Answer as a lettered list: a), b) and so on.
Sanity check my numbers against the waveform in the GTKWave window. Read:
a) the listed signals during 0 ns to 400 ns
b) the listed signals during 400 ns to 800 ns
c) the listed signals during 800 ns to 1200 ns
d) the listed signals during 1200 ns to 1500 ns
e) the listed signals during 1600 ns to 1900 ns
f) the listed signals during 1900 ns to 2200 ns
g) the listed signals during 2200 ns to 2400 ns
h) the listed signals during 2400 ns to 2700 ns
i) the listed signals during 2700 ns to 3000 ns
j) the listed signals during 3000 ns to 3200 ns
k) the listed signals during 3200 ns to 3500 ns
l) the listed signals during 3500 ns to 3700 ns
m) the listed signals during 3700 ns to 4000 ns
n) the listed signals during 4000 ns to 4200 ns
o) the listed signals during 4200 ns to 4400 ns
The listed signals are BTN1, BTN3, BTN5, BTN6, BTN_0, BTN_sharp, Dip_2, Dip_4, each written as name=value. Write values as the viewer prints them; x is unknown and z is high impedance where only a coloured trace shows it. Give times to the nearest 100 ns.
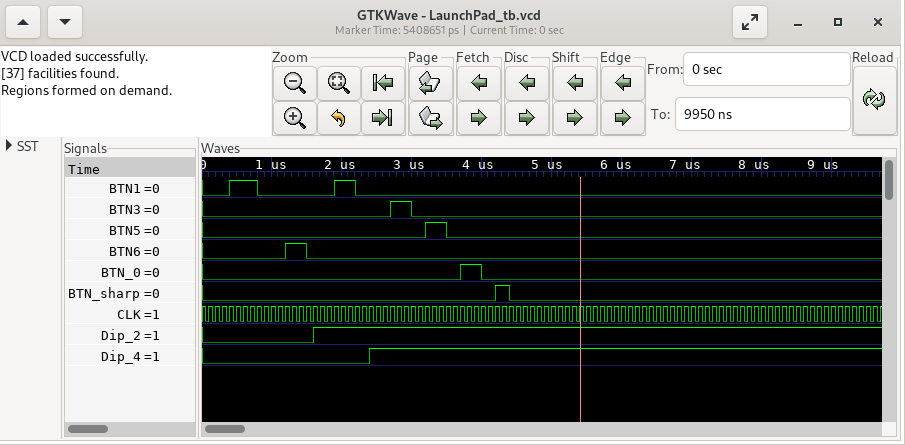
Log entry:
a) BTN1=0, BTN3=0, BTN5=0, BTN6=0, BTN_0=0, BTN_sharp=0, Dip_2=0, Dip_4=0
b) BTN1=1, BTN3=0, BTN5=0, BTN6=0, BTN_0=0, BTN_sharp=0, Dip_2=0, Dip_4=0
c) BTN1=0, BTN3=0, BTN5=0, BTN6=0, BTN_0=0, BTN_sharp=0, Dip_2=0, Dip_4=0
d) BTN1=0, BTN3=0, BTN5=0, BTN6=1, BTN_0=0, BTN_sharp=0, Dip_2=0, Dip_4=0
e) BTN1=0, BTN3=0, BTN5=0, BTN6=0, BTN_0=0, BTN_sharp=0, Dip_2=1, Dip_4=0
f) BTN1=1, BTN3=0, BTN5=0, BTN6=0, BTN_0=0, BTN_sharp=0, Dip_2=1, Dip_4=0
g) BTN1=0, BTN3=0, BTN5=0, BTN6=0, BTN_0=0, BTN_sharp=0, Dip_2=1, Dip_4=0
h) BTN1=0, BTN3=0, BTN5=0, BTN6=0, BTN_0=0, BTN_sharp=0, Dip_2=1, Dip_4=1
i) BTN1=0, BTN3=1, BTN5=0, BTN6=0, BTN_0=0, BTN_sharp=0, Dip_2=1, Dip_4=1
j) BTN1=0, BTN3=0, BTN5=0, BTN6=0, BTN_0=0, BTN_sharp=0, Dip_2=1, Dip_4=1
k) BTN1=0, BTN3=0, BTN5=1, BTN6=0, BTN_0=0, BTN_sharp=0, Dip_2=1, Dip_4=1
l) BTN1=0, BTN3=0, BTN5=0, BTN6=0, BTN_0=0, BTN_sharp=0, Dip_2=1, Dip_4=1
m) BTN1=0, BTN3=0, BTN5=0, BTN6=0, BTN_0=1, BTN_sharp=0, Dip_2=1, Dip_4=1
n) BTN1=0, BTN3=0, BTN5=0, BTN6=0, BTN_0=0, BTN_sharp=0, Dip_2=1, Dip_4=1
o) BTN1=0, BTN3=0, BTN5=0, BTN6=0, BTN_0=0, BTN_sharp=1, Dip_2=1, Dip_4=1
